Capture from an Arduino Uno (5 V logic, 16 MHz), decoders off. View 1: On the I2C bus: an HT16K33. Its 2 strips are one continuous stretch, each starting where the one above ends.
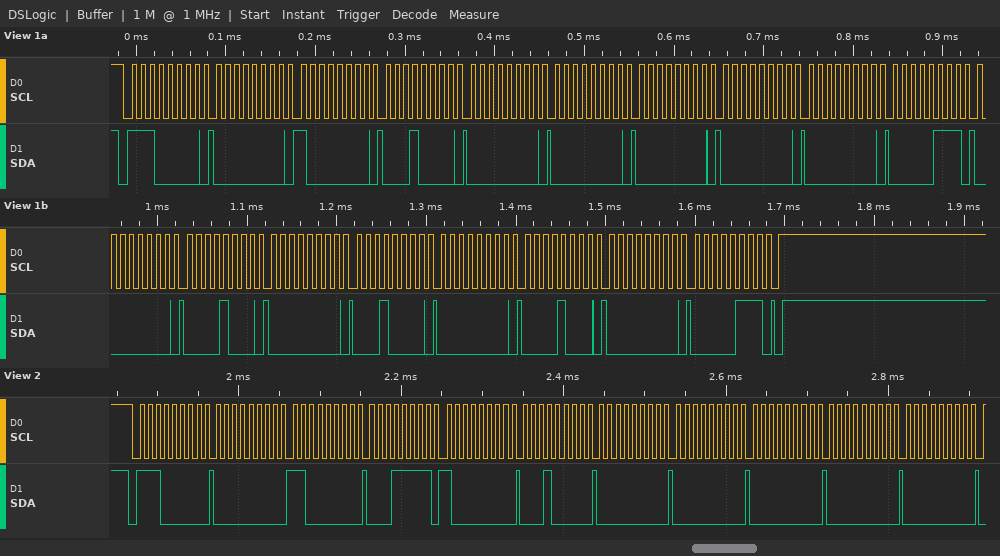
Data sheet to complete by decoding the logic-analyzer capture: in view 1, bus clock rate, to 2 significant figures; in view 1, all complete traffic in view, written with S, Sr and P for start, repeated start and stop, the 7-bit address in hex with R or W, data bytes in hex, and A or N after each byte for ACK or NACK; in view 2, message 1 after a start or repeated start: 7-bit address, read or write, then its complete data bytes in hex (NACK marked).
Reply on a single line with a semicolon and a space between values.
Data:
100 kHz; S 70W A 00 A 80 A 10 A 00 A 00 A 00 A 00 A 00 A 07 A 00 A 08 A 00 A 10 A 00 A 08 A 00 A 07 A P; 0x70 write: 00 C0 1F 80 10 00 00 00 00 00
